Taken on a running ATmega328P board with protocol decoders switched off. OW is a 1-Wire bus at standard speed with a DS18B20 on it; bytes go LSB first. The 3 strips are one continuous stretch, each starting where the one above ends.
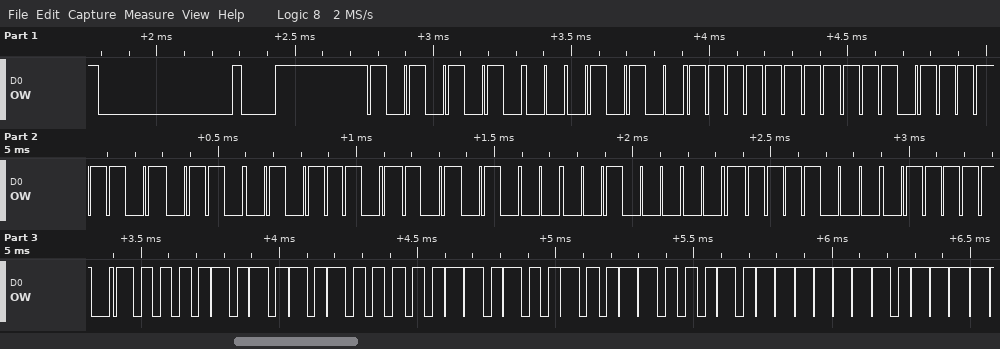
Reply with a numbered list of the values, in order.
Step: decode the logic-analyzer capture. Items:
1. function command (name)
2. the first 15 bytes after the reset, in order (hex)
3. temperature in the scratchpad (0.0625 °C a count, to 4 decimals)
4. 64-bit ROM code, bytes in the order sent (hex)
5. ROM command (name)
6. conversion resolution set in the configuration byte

1. Read Scratchpad
2. 55 28 FF F7 6B BA 15 04 1F BE 50 05 4B 46 7F
3. 85.0000 °C
4. 28 FF F7 6B BA 15 04 1F
5. Match ROM
6. 12 bits
